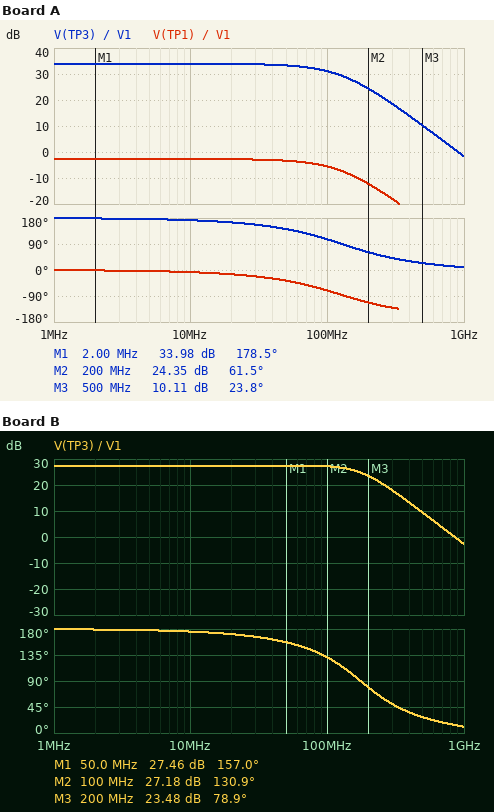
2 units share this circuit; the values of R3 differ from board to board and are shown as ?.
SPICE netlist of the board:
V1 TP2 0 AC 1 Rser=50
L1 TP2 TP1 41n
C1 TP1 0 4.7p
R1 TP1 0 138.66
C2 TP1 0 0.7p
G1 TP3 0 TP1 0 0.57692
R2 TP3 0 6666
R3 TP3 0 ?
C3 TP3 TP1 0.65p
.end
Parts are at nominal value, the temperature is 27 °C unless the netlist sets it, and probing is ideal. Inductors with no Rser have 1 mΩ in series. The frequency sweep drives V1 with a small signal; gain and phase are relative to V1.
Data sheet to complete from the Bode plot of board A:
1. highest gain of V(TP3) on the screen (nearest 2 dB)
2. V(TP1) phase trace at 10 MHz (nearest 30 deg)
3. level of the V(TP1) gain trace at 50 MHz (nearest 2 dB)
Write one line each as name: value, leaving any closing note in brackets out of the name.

highest gain of V(TP3) on the screen: 34 dB
V(TP1) phase trace at 10 MHz: 0 deg
level of the V(TP1) gain trace at 50 MHz: -4 dB
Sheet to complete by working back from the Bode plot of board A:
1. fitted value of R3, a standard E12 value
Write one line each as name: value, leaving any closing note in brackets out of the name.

fitted value of R3, a standard E12 value: 120 Ω
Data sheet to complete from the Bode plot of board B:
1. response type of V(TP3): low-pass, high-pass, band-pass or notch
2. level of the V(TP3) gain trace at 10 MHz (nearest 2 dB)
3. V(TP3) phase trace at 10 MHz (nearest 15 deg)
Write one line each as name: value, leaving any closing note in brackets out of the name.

response type of V(TP3): low-pass, high-pass, band-pass or notch: low-pass
level of the V(TP3) gain trace at 10 MHz: 28 dB
V(TP3) phase trace at 10 MHz: 180 deg
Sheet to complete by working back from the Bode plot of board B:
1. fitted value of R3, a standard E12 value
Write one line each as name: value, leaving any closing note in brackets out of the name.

fitted value of R3, a standard E12 value: 56 Ω
